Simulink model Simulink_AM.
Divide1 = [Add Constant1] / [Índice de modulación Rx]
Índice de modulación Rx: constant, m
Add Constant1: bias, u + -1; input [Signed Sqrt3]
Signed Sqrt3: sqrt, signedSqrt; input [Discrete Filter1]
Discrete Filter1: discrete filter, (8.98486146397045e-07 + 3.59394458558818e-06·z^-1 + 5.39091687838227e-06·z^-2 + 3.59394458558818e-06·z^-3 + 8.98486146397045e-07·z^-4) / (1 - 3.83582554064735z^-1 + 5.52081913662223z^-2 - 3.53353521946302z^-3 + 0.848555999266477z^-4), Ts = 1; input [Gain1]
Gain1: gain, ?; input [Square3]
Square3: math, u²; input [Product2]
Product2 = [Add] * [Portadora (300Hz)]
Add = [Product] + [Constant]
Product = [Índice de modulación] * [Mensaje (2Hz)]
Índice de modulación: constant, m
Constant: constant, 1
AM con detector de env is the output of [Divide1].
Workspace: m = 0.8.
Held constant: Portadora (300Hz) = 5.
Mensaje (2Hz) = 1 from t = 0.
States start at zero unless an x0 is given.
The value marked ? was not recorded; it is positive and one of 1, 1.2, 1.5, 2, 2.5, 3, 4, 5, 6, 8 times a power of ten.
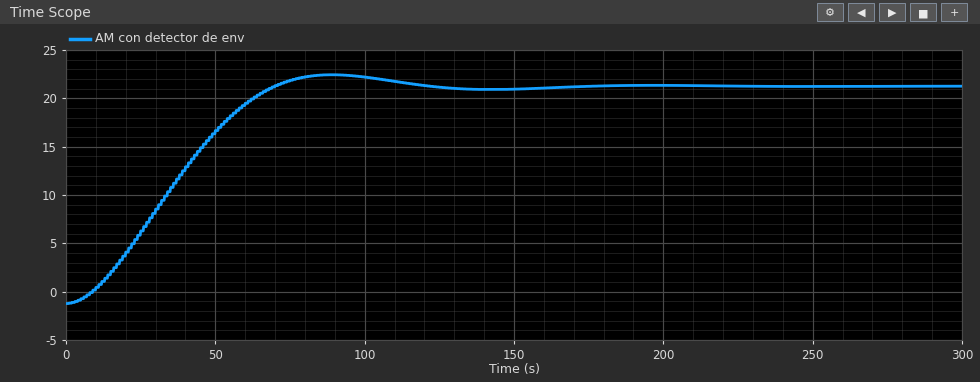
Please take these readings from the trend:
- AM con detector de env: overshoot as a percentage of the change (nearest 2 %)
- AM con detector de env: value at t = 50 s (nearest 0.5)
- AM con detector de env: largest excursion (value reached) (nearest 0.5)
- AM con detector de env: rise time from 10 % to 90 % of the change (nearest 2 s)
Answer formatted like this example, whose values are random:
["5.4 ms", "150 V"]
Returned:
["6 %", "16.5", "22.5", "46 s"]
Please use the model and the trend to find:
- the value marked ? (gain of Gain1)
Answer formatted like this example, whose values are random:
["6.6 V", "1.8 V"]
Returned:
["4"]
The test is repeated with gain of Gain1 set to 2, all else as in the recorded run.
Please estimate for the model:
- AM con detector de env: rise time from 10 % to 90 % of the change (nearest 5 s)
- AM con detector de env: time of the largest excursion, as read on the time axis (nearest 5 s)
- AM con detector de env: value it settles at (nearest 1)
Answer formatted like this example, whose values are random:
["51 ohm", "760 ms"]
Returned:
["45 s", "90 s", "15"]
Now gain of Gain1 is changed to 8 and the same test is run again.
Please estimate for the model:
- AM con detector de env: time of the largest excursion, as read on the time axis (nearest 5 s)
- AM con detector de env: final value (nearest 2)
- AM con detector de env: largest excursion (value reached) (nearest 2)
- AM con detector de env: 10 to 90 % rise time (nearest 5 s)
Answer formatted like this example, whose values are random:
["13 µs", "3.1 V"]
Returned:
["90 s", "30", "32", "45 s"]
